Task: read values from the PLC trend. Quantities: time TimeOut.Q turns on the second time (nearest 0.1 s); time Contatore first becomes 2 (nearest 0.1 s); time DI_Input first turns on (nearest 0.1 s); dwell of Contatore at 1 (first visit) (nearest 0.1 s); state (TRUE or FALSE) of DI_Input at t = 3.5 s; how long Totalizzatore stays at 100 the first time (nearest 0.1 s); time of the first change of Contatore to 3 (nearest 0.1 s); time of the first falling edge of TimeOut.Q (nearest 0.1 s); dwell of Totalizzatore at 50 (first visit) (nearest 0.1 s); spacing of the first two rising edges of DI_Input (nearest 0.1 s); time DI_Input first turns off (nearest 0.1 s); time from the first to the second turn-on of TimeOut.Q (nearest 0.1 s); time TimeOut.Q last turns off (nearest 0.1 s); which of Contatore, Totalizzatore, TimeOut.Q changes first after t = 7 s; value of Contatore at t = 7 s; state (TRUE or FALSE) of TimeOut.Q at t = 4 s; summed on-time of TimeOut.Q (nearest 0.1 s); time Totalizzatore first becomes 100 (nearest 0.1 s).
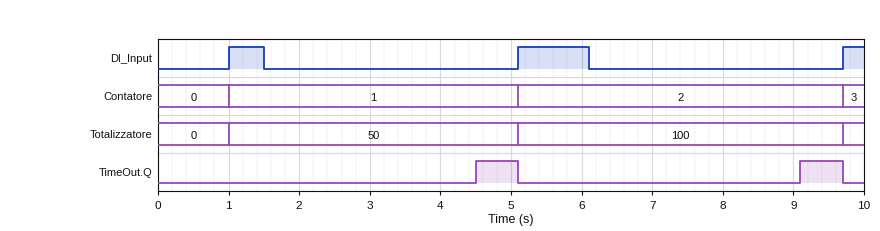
9.1 s
5.1 s
1.0 s
4.1 s
FALSE
4.6 s
9.7 s
5.1 s
4.1 s
4.1 s
1.5 s
4.6 s
9.7 s
TimeOut.Q
2
FALSE
1.2 s
5.1 s
